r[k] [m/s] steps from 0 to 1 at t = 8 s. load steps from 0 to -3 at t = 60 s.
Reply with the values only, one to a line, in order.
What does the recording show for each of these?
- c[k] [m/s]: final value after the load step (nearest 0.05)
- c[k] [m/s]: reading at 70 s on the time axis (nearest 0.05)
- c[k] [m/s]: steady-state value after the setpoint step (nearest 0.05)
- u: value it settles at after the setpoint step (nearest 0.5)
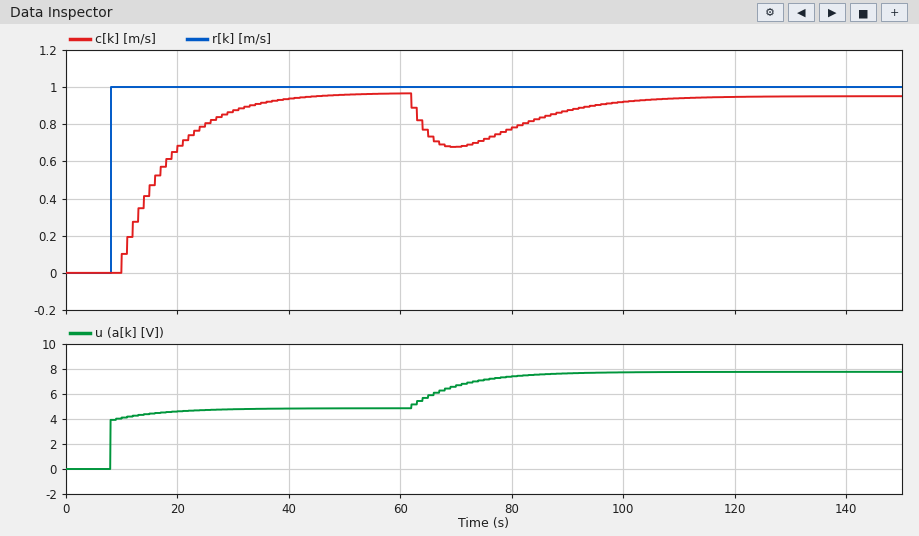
0.95
0.70
0.95
5.0
